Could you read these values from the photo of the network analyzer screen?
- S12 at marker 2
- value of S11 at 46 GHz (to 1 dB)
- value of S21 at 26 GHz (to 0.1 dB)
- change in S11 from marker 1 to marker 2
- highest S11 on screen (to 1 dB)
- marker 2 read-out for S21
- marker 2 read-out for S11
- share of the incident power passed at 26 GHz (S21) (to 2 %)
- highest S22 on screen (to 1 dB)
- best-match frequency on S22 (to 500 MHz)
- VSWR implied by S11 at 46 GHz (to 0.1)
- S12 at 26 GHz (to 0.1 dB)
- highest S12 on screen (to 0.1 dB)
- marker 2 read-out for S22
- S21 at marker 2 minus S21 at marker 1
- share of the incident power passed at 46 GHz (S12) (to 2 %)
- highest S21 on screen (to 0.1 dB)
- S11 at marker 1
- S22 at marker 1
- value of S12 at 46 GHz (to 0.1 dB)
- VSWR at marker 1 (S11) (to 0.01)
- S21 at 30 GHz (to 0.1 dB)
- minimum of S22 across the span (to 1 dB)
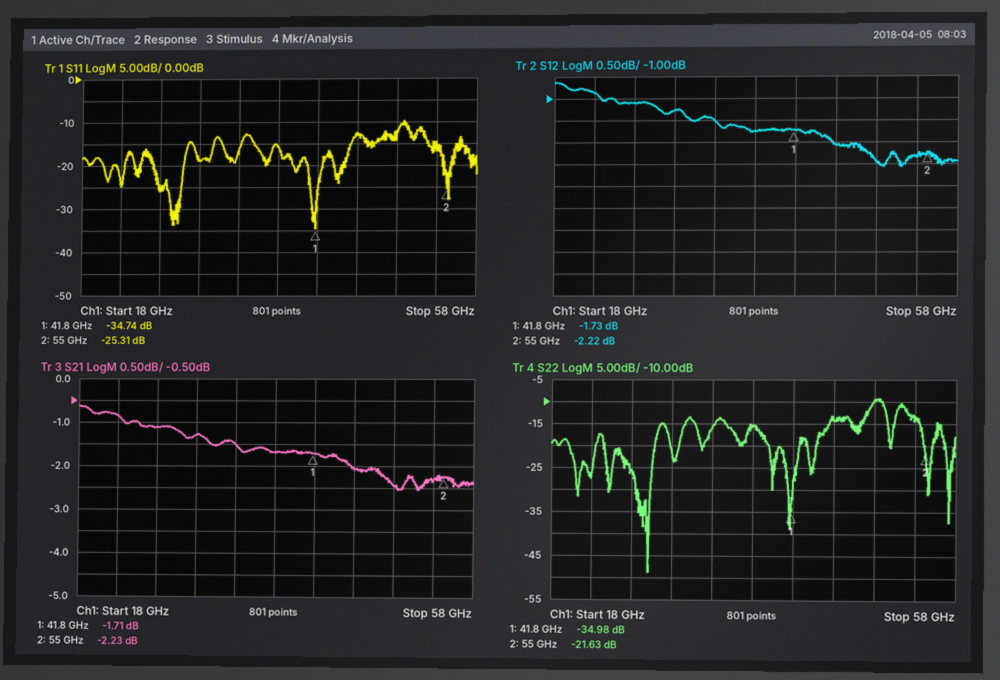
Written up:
-2.22 dB
-13 dB
-1.1 dB
9.43 dB
-10 dB
-2.23 dB
-25.31 dB
78 %
-9 dB
27.5 GHz
1.6
-1.1 dB
-0.6 dB
-21.63 dB
-0.52 dB
62 %
-0.6 dB
-34.74 dB
-34.98 dB
-2.1 dB
1.04
-1.3 dB
-49 dB
